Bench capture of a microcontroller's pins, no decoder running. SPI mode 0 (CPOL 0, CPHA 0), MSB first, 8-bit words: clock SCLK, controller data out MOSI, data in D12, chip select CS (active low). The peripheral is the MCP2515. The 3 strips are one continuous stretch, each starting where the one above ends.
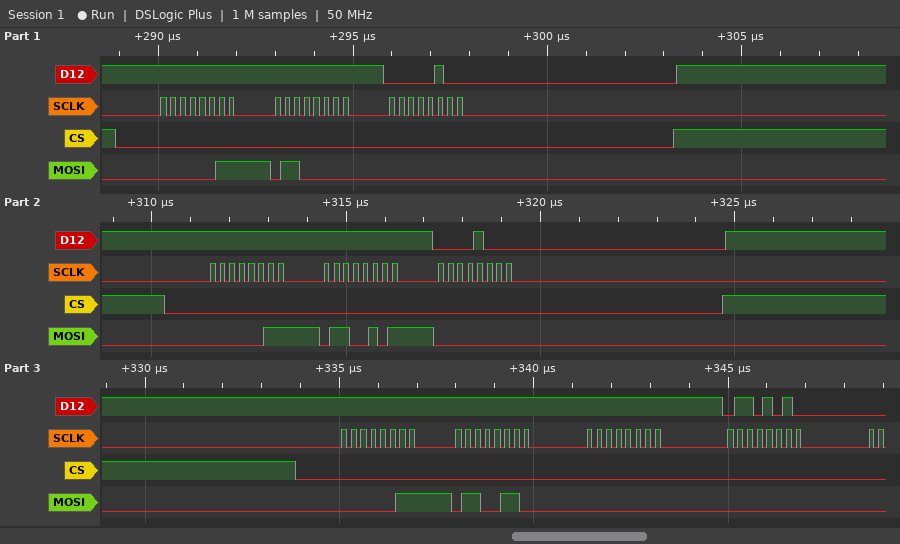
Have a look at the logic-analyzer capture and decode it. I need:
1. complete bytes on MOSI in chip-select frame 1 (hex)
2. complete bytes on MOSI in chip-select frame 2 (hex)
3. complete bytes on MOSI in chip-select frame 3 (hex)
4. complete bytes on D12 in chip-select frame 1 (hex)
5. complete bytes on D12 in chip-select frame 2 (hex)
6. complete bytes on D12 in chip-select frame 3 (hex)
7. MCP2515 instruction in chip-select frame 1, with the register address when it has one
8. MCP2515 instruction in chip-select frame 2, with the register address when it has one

03 60 00
03 65 00
03 66 00 00
FF FF 04
FF FF 08
FF FF FF 6A
READ 0x60
READ 0x65
